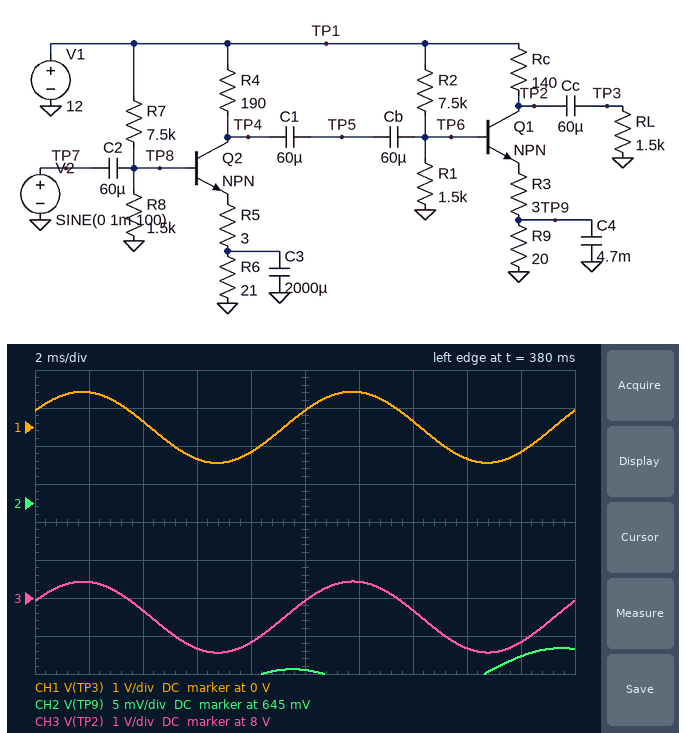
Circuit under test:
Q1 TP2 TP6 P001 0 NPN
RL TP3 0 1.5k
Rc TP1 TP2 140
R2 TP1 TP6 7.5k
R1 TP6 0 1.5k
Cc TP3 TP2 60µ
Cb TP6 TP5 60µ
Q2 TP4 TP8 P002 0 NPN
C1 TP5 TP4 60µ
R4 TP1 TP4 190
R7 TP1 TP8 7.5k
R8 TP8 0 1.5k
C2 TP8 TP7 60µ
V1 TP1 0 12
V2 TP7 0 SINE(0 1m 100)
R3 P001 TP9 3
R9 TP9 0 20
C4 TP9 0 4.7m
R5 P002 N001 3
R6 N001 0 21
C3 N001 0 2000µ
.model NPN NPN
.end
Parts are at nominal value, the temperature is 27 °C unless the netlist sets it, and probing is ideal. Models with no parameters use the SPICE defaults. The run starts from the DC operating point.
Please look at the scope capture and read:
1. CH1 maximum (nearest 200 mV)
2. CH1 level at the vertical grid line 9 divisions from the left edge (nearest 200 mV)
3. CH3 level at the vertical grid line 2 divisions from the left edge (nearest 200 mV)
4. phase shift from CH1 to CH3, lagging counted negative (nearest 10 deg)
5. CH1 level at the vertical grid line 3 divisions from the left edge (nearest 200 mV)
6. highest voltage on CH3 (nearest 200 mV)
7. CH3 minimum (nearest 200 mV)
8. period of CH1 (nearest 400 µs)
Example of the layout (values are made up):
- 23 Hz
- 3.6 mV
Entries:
- 1.0 V
- -600 mV
- 7.6 V
- 0 deg
- -800 mV
- 8.4 V
- 6.6 V
- 10.0 ms
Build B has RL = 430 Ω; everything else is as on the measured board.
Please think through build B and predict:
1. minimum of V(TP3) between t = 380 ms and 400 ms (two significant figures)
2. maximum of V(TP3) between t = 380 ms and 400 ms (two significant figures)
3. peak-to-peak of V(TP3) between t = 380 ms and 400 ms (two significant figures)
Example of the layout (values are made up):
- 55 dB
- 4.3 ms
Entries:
- -760 mV
- 780 mV
- 1.5 V
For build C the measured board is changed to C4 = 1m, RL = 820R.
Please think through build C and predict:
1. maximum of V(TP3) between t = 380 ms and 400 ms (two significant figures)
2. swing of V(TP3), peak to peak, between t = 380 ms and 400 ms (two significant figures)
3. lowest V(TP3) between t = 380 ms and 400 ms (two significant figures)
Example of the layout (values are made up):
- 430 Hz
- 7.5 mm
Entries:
- 710 mV
- 1.6 V
- -920 mV
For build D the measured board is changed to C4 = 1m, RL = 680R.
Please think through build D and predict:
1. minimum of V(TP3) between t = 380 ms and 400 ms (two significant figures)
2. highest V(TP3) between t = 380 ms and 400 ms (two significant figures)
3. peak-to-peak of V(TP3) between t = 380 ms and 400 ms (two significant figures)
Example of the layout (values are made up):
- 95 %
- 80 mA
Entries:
- -870 mV
- 710 mV
- 1.6 V
